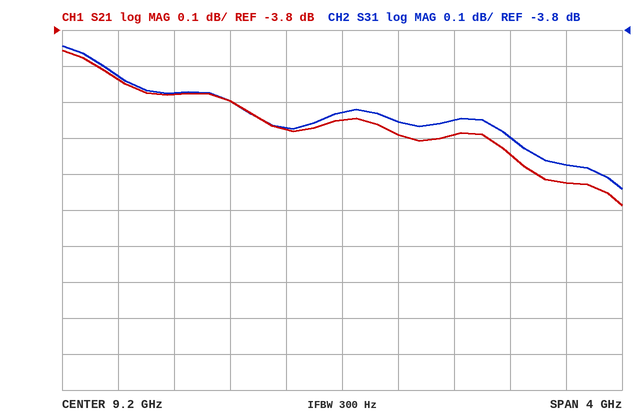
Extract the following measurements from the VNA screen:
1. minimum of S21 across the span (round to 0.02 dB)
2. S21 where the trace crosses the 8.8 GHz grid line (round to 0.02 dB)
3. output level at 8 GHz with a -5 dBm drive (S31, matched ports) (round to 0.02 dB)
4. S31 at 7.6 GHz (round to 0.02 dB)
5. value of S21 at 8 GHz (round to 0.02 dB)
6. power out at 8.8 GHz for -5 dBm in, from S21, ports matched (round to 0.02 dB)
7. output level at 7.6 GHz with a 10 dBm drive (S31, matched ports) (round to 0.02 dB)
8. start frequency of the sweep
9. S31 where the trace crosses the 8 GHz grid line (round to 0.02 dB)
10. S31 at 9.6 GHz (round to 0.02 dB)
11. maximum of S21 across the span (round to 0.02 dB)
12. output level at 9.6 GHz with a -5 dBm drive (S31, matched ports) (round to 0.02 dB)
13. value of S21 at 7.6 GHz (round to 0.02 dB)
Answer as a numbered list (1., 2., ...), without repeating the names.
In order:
1. -4.28 dB
2. -4.08 dB
3. -8.98 dBm
4. -3.92 dB
5. -3.98 dB
6. -9.08 dBm
7. 6.08 dBm
8. 7.2 GHz
9. -3.98 dB
10. -4.06 dB
11. -3.86 dB
12. -9.06 dBm
13. -3.94 dB
